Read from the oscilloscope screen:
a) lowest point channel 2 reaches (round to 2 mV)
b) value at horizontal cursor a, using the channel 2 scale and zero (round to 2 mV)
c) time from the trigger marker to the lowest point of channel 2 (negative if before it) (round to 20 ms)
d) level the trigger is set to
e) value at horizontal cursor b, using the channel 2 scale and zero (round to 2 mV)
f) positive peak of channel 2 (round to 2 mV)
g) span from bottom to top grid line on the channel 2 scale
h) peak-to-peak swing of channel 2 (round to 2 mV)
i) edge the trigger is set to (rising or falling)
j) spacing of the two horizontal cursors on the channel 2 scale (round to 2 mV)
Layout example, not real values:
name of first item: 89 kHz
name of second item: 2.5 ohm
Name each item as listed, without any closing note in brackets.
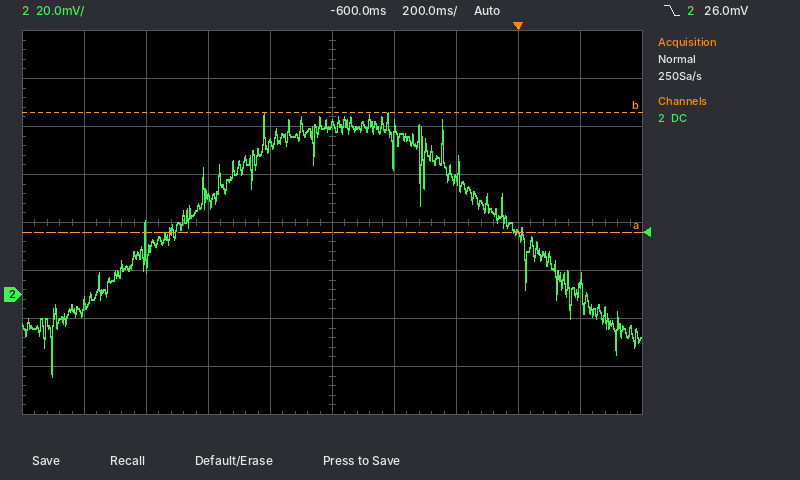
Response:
lowest point channel 2 reaches: -34 mV
value at horizontal cursor a, using the channel 2 scale and zero: 26 mV
time from the trigger marker to the lowest point of channel 2 (negative if before it): -1.50 s
level the trigger is set to: 26.0 mV
value at horizontal cursor b, using the channel 2 scale and zero: 76 mV
positive peak of channel 2: 76 mV
span from bottom to top grid line on the channel 2 scale: 160 mV
peak-to-peak swing of channel 2: 110 mV
edge the trigger is set to: falling
spacing of the two horizontal cursors on the channel 2 scale: 50 mV
